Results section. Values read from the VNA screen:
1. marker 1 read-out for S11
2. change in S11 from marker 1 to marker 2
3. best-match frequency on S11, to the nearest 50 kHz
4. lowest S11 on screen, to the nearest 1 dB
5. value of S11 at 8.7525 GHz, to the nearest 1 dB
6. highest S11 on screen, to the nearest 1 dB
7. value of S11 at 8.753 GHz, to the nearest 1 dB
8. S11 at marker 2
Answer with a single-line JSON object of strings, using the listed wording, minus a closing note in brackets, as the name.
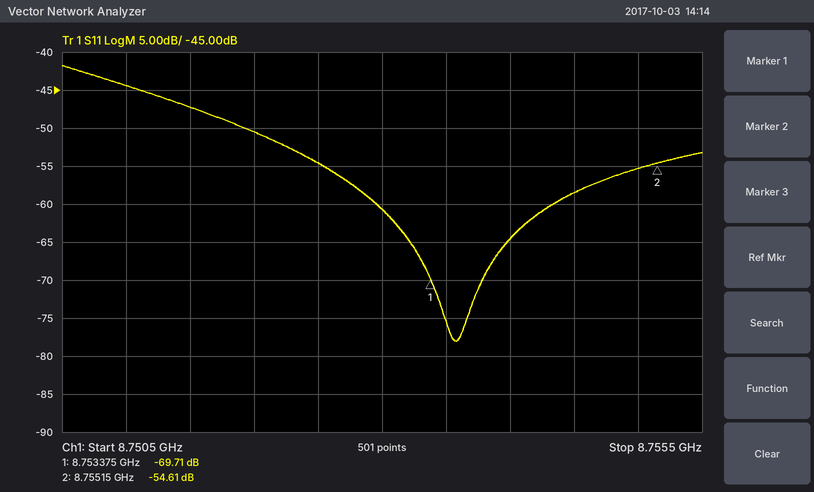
{"marker 1 read-out for S11": "-69.71 dB", "change in S11 from marker 1 to marker 2": "15.10 dB", "best-match frequency on S11, to the nearest 50 kHz": "8.75360 GHz", "lowest S11 on screen, to the nearest 1 dB": "-78 dB", "value of S11 at 8.7525 GHz, to the nearest 1 dB": "-55 dB", "highest S11 on screen, to the nearest 1 dB": "-42 dB", "value of S11 at 8.753 GHz, to the nearest 1 dB": "-61 dB", "S11 at marker 2": "-54.61 dB"}
